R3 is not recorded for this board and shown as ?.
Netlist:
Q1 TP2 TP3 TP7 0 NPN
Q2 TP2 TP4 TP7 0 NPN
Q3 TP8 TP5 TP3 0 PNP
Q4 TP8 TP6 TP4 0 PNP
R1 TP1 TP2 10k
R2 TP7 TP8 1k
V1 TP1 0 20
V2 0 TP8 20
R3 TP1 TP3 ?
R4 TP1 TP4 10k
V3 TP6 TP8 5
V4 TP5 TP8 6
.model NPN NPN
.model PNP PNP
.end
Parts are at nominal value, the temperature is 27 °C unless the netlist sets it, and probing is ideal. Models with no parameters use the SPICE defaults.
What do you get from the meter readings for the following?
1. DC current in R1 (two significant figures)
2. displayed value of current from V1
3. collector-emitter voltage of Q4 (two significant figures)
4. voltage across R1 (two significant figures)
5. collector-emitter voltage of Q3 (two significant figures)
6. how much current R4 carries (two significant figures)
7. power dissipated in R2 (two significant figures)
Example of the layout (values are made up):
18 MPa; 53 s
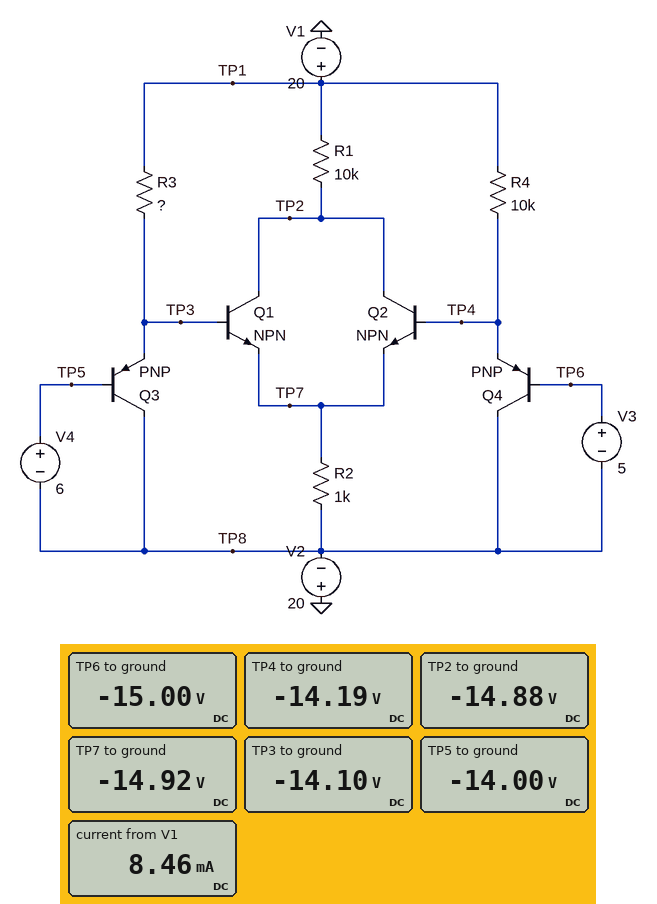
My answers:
3.5 mA; 8.46 mA; -5.8 V; 35 V; -5.9 V; 3.4 mA; 26 mW
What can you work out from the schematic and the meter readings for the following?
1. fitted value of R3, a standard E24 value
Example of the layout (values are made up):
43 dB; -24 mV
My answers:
22 kΩ
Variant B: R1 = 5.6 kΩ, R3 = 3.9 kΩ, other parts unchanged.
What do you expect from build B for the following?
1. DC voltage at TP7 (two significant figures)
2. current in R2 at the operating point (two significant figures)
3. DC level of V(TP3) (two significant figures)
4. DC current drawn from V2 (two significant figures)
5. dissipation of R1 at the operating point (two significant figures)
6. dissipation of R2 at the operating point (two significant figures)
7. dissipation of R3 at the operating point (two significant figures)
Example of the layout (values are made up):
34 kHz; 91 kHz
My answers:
-14 V; 6.0 mA; -13 V; 18 mA; 200 mW; 36 mW; 280 mW
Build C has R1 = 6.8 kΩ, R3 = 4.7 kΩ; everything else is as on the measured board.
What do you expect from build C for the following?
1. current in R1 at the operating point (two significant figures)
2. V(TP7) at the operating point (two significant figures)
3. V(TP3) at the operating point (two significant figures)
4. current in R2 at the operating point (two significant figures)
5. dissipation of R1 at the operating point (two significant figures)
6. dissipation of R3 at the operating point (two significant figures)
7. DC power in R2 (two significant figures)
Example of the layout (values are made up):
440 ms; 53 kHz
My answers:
5.0 mA; -14 V; -13 V; 6.0 mA; 170 mW; 230 mW; 36 mW
